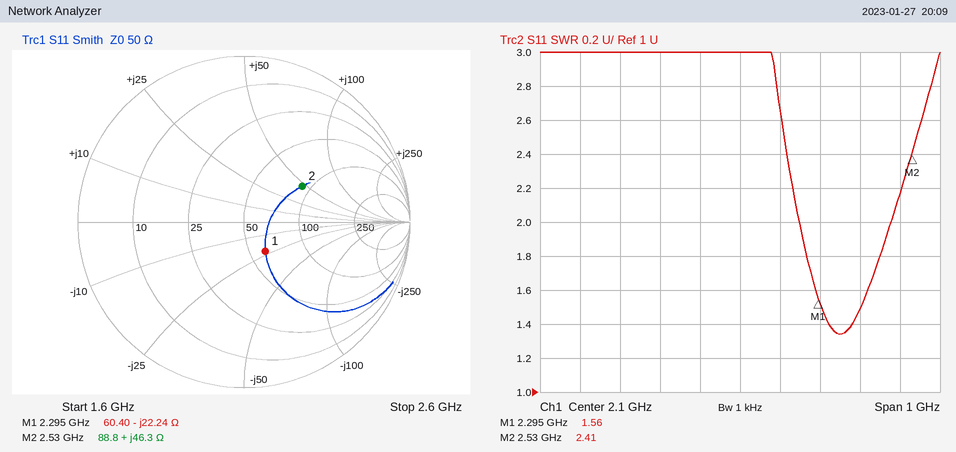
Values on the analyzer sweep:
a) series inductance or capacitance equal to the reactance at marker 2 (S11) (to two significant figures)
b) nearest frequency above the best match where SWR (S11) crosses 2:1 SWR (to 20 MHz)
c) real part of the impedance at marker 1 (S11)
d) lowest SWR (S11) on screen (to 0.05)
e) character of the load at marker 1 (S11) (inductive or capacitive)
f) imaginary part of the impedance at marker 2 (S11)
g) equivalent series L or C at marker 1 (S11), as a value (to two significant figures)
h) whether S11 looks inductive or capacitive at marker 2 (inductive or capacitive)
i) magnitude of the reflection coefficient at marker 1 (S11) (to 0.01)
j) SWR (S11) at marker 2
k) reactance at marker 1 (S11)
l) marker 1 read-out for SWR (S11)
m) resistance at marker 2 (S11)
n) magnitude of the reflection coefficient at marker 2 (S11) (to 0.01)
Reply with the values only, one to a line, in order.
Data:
2.9 nH
2.48 GHz
60.40 Ω
1.35
capacitive
+46.3 Ω
3.1 pF
inductive
0.22
2.41
-22.24 Ω
1.56
88.8 Ω
0.41
